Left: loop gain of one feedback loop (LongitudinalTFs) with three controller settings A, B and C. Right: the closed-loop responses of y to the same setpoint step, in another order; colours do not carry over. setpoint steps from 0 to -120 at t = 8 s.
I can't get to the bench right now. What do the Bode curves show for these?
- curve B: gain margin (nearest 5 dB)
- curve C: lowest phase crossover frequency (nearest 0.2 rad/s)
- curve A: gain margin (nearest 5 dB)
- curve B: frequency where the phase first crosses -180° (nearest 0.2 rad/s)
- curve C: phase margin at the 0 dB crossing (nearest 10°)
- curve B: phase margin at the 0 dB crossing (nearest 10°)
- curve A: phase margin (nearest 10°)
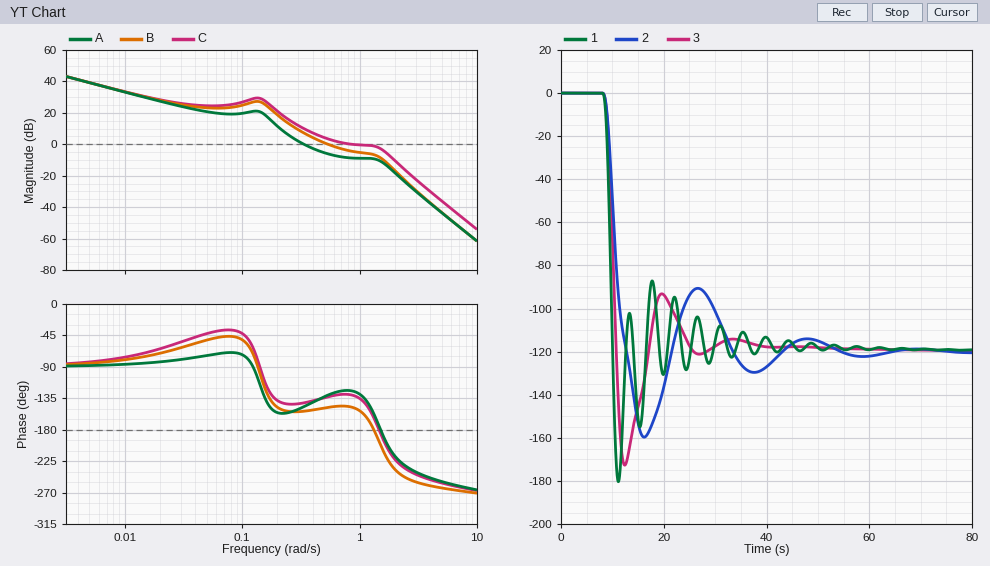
5 dB
1.4 rad/s
10 dB
1.4 rad/s
50°
30°
30°
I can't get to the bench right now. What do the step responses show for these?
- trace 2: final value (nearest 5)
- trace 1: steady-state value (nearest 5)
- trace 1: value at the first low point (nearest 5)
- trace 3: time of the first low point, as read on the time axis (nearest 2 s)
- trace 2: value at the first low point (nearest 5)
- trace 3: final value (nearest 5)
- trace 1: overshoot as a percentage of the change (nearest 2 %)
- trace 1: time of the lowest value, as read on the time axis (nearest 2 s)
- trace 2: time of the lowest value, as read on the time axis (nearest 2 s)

-120
-120
-180
12 s
-160
-120
50 %
12 s
16 s
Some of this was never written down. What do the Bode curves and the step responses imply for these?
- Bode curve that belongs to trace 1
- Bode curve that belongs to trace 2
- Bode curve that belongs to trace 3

C
A
B
